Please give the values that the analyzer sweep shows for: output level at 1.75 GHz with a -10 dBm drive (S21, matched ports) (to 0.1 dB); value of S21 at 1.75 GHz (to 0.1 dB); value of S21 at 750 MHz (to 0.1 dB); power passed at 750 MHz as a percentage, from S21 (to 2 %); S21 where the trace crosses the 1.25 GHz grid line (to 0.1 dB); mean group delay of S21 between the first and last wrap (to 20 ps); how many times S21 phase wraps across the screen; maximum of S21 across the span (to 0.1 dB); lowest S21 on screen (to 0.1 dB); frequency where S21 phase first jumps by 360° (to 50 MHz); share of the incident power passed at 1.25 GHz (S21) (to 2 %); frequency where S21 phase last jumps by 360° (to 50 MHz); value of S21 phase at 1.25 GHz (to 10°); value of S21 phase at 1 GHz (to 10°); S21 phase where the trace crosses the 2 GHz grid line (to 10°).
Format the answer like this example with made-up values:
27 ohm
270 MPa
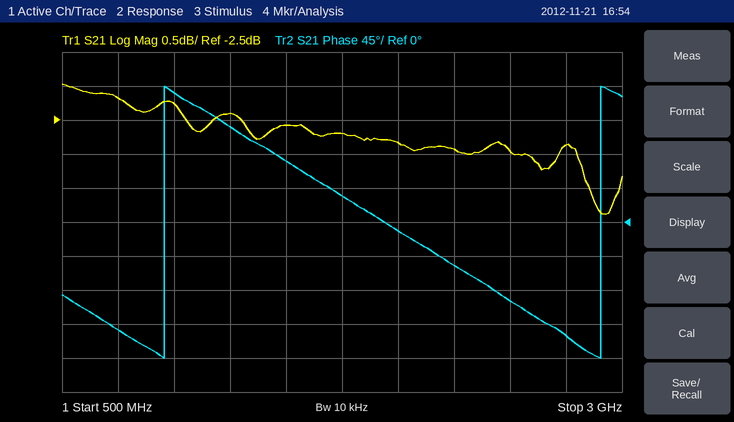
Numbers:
-12.7 dBm
-2.7 dB
-2.2 dB
60 %
-2.4 dB
520 ps
2
-2.0 dB
-3.9 dB
950 MHz
58 %
2.90 GHz
130°
170°
-10°
